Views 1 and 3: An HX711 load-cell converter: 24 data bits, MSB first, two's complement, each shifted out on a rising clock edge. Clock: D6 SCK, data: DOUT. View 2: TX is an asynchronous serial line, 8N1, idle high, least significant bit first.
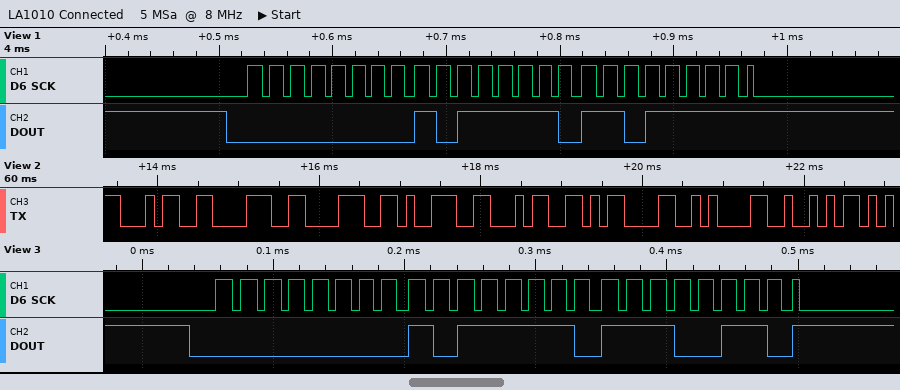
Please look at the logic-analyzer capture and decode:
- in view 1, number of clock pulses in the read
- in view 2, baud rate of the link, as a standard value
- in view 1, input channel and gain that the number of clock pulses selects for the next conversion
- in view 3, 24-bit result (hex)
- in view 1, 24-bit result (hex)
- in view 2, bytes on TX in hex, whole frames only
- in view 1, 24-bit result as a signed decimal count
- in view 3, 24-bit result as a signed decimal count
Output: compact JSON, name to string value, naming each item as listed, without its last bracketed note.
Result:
{"in view 1, number of clock pulses in the read": "25", "in view 2, baud rate of the link, as a standard value": "9600 baud", "in view 1, input channel and gain that the number of clock pulses selects for the next conversion": "channel A, gain 128", "in view 3, 24-bit result": "0x00BEE6", "in view 1, 24-bit result": "0x00BEDF", "in view 2, bytes on TX in hex, whole frames only": "0x34 0x38 0x38 0x39 0x34 0x0D 0x0A 0x52", "in view 1, 24-bit result as a signed decimal count": "48863", "in view 3, 24-bit result as a signed decimal count": "48870"}
